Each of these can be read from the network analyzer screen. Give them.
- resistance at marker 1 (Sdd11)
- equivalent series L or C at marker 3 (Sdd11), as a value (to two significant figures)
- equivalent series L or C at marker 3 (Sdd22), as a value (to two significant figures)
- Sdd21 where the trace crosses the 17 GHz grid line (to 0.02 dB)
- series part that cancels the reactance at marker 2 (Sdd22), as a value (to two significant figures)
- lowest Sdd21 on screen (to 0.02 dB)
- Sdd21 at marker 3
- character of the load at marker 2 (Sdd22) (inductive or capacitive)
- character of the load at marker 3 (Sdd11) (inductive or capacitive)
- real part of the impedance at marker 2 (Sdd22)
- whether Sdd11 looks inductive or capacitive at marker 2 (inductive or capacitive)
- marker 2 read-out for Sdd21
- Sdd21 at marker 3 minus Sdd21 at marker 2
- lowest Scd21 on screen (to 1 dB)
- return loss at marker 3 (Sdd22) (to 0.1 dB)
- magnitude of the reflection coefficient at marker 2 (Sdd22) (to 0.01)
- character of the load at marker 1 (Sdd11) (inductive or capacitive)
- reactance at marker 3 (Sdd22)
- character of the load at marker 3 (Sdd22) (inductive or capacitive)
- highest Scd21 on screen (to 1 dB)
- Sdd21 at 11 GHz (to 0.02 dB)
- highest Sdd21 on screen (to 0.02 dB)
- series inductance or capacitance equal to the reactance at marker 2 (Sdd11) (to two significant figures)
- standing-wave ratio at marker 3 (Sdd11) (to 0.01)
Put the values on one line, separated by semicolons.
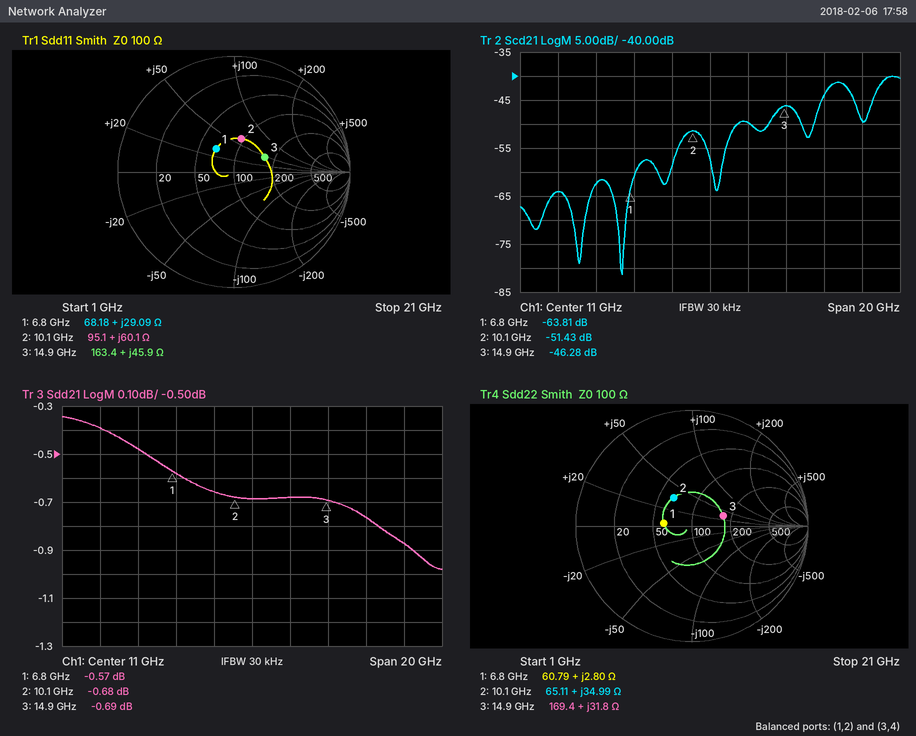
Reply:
68.18 Ω; 490 pH; 340 pH; -0.76 dB; 450 fF; -0.98 dB; -0.69 dB; inductive; inductive; 65.11 Ω; inductive; -0.68 dB; -0.01 dB; -81 dB; 11.0 dB; 0.29; inductive; +31.8 Ω; inductive; -40 dB; -0.68 dB; -0.34 dB; 950 pH; 1.83
